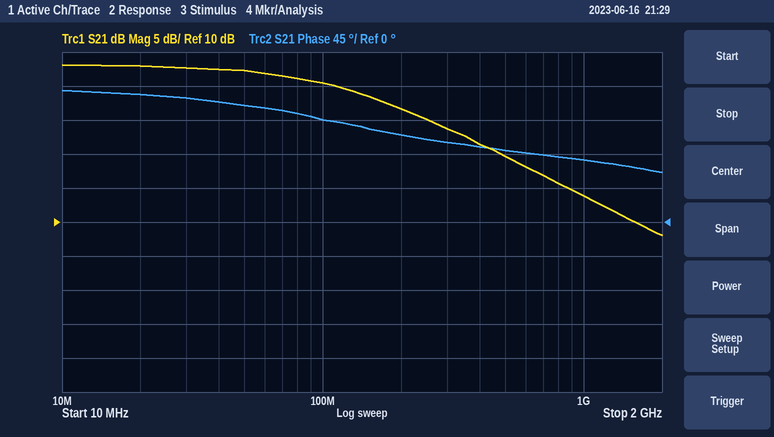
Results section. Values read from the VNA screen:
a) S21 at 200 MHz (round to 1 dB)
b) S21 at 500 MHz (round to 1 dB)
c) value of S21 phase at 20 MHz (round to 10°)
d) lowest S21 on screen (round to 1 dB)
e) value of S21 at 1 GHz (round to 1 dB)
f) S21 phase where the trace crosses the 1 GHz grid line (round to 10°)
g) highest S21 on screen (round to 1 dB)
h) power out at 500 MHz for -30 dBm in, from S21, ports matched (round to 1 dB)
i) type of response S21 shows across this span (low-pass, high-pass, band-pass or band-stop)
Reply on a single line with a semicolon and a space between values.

27 dB; 20 dB; 170°; 8 dB; 14 dB; 80°; 33 dB; -10 dBm; low-pass
